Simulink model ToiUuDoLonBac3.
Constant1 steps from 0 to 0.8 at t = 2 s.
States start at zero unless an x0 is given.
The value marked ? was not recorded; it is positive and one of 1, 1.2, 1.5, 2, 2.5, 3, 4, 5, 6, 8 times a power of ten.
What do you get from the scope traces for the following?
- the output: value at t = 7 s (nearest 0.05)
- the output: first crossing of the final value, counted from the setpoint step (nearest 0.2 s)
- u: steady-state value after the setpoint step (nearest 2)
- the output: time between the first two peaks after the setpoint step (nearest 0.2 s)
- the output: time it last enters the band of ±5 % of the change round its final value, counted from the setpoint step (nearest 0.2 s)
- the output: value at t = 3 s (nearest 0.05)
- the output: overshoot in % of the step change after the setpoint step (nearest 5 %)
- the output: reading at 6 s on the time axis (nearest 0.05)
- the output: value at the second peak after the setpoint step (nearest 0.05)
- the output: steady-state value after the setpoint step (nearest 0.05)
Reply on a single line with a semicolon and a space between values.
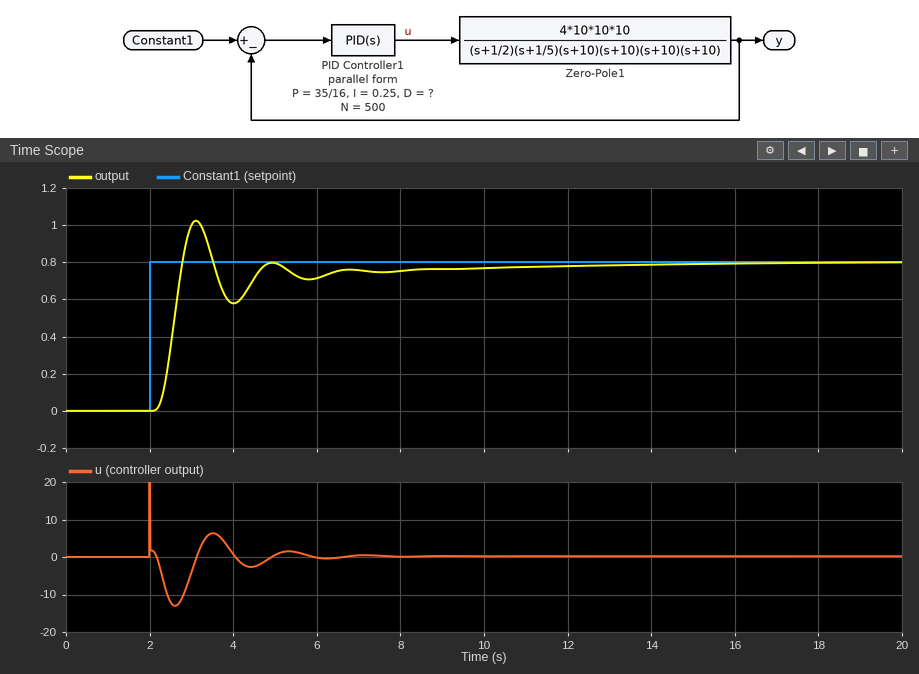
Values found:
0.75; 0.8 s; 0; 1.8 s; 6.4 s; 1.00; 30 %; 0.70; 0.80; 0.80
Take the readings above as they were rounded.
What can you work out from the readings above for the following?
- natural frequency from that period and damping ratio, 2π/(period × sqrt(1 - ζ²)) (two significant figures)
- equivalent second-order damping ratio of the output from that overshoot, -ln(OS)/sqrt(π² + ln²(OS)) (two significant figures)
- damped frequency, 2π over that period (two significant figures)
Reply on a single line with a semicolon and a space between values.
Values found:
3.7 rad/s; 0.36; 3.5 rad/s
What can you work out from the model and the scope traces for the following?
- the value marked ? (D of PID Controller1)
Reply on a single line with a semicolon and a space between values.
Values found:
8
